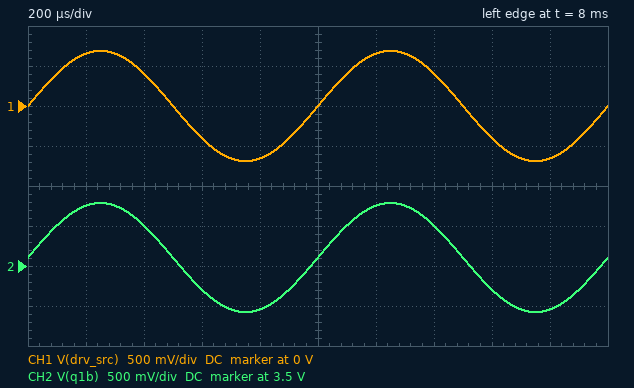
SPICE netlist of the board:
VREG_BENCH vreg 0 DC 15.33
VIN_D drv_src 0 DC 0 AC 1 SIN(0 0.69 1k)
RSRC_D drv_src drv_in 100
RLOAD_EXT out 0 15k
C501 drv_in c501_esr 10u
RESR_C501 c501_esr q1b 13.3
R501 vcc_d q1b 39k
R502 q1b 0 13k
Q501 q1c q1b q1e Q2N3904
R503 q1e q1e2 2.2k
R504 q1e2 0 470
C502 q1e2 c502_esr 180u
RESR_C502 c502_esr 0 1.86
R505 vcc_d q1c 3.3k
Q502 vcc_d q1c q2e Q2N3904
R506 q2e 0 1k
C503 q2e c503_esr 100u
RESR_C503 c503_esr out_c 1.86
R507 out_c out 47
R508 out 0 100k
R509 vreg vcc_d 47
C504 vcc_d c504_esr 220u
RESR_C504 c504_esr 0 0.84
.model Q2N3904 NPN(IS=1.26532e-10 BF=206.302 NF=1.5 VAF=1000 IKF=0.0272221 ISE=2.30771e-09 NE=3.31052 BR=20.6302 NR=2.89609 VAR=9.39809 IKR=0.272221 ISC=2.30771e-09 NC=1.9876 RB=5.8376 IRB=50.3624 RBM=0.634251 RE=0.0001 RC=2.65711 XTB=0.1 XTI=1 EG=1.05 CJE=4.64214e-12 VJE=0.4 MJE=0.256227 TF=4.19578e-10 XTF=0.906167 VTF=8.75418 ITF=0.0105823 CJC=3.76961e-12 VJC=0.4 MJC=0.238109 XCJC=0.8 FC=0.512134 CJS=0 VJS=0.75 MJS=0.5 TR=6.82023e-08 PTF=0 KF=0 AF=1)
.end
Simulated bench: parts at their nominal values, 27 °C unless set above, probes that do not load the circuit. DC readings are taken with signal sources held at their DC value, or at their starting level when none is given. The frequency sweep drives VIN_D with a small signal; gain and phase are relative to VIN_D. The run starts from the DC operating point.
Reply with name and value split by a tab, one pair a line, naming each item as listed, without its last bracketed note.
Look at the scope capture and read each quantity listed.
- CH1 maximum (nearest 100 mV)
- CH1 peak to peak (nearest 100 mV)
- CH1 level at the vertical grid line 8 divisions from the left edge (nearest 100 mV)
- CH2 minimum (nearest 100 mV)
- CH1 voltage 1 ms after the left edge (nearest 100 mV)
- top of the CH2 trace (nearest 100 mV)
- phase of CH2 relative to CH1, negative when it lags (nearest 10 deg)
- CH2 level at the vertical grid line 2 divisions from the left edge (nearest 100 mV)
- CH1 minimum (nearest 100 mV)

CH1 maximum	700 mV
CH1 peak to peak	1.4 V
CH1 level at the vertical grid line 8 divisions from the left edge	-400 mV
CH2 minimum	2.9 V
CH1 voltage 1 ms after the left edge	0 V
top of the CH2 trace	4.3 V
phase of CH2 relative to CH1, negative when it lags	0 deg
CH2 level at the vertical grid line 2 divisions from the left edge	4.0 V
CH1 minimum	-700 mV
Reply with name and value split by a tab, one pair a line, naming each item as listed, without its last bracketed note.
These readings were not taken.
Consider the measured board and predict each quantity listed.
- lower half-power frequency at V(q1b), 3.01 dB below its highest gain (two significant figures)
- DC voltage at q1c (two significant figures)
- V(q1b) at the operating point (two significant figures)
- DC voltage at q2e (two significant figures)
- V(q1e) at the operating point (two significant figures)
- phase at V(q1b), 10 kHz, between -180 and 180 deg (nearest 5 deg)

lower half-power frequency at V(q1b), 3.01 dB below its highest gain	1.6 Hz
DC voltage at q1c	11 V
V(q1b) at the operating point	3.6 V
DC voltage at q2e	10 V
V(q1e) at the operating point	3.0 V
phase at V(q1b), 10 kHz, between -180 and 180 deg	0 deg
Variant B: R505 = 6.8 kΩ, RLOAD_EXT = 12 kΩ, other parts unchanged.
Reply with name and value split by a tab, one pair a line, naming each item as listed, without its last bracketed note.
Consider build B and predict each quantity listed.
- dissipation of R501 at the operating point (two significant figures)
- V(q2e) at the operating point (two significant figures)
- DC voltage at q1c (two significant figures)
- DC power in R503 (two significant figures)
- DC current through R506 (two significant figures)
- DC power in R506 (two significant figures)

dissipation of R501 at the operating point	3.3 mW
V(q2e) at the operating point	6.3 V
DC voltage at q1c	7.0 V
DC power in R503	2.8 mW
DC current through R506	6.3 mA
DC power in R506	40 mW
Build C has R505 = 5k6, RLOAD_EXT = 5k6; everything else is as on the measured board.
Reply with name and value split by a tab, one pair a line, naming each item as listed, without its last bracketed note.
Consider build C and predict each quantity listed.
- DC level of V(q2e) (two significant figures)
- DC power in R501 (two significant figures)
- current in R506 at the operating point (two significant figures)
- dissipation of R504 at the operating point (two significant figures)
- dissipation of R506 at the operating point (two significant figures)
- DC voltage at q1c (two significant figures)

DC level of V(q2e)	7.6 V
DC power in R501	3.3 mW
current in R506 at the operating point	7.6 mA
dissipation of R504 at the operating point	600 µW
dissipation of R506 at the operating point	58 mW
DC voltage at q1c	8.3 V
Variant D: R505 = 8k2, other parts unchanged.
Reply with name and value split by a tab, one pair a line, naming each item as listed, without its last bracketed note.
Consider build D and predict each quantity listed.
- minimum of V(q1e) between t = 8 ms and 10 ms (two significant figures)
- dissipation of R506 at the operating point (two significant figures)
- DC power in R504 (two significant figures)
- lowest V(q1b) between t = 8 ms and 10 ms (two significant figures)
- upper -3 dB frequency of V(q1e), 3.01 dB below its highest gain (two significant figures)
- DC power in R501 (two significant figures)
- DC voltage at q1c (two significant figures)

minimum of V(q1e) between t = 8 ms and 10 ms	2.4 V
dissipation of R506 at the operating point	23 mW
DC power in R504	610 µW
lowest V(q1b) between t = 8 ms and 10 ms	3.0 V
upper -3 dB frequency of V(q1e), 3.01 dB below its highest gain	1.1 GHz
DC power in R501	3.3 mW
DC voltage at q1c	5.5 V
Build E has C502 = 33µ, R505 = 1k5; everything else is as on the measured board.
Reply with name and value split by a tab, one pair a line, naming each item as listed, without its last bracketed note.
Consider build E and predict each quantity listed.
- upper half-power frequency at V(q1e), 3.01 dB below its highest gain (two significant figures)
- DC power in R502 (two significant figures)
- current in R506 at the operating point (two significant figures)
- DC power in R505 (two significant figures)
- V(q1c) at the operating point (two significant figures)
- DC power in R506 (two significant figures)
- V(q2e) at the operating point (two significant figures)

upper half-power frequency at V(q1e), 3.01 dB below its highest gain	1.1 GHz
DC power in R502	990 µW
current in R506 at the operating point	12 mA
DC power in R505	2.2 mW
V(q1c) at the operating point	13 V
DC power in R506	150 mW
V(q2e) at the operating point	12 V
